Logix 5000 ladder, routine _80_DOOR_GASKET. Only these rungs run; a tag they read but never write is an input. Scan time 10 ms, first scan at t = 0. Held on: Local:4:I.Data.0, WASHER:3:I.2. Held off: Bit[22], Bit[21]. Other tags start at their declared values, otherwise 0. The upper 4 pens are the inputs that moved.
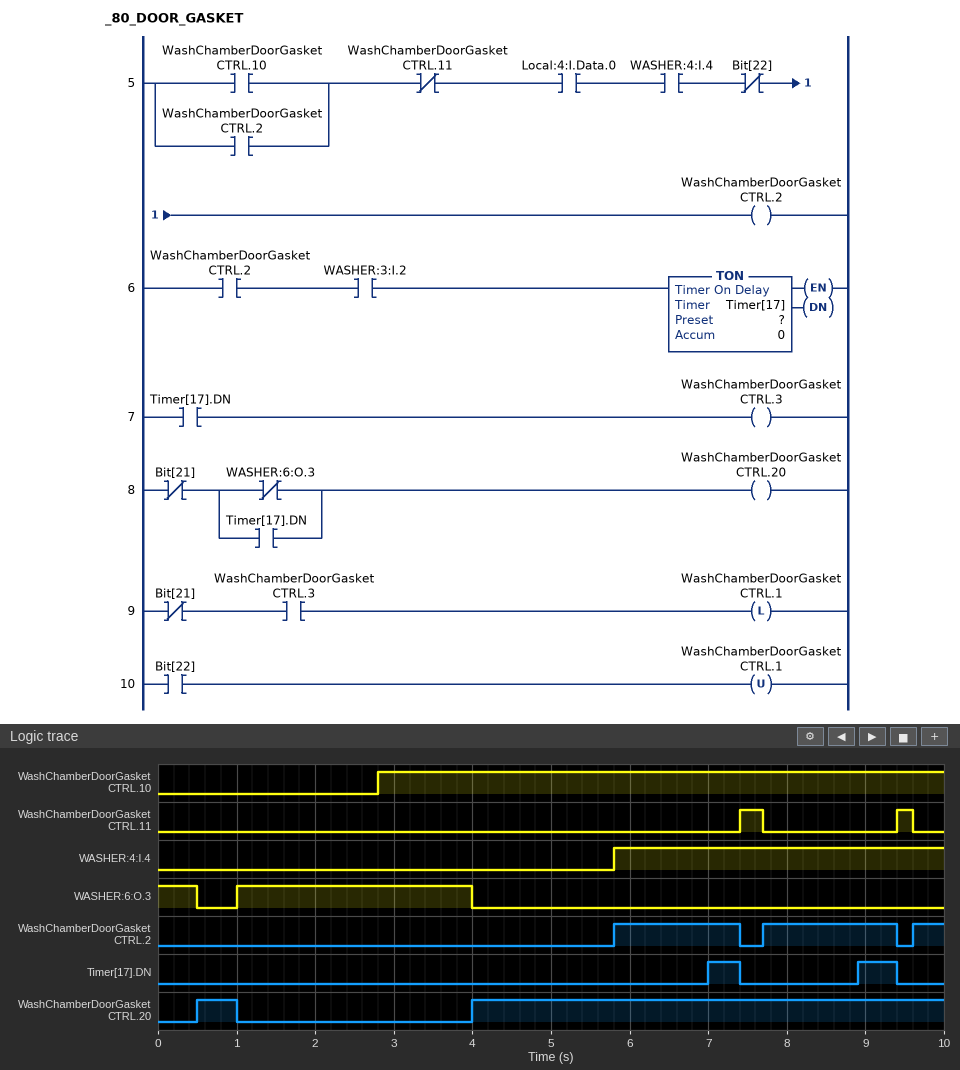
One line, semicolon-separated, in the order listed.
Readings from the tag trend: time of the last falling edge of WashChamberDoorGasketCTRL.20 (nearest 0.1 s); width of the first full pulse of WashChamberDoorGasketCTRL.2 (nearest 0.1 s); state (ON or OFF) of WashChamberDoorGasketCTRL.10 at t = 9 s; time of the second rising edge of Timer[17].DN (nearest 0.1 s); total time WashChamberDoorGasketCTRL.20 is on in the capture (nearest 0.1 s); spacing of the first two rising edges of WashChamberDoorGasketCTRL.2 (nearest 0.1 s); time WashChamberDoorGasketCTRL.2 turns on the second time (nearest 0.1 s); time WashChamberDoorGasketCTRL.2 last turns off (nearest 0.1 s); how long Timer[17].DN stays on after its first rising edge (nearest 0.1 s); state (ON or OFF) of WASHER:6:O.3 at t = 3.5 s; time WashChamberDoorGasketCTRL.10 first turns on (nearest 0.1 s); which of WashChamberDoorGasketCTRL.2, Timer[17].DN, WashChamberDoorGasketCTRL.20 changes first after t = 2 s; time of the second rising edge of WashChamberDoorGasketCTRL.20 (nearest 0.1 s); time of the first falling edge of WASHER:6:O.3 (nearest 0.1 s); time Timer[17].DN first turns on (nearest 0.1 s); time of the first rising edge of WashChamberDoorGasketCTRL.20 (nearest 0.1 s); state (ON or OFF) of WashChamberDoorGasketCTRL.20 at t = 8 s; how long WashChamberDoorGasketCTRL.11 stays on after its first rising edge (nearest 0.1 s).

1.0 s; 1.6 s; ON; 8.9 s; 6.5 s; 1.9 s; 7.7 s; 9.4 s; 0.4 s; ON; 2.8 s; WashChamberDoorGasketCTRL.20; 4.0 s; 0.5 s; 7.0 s; 0.5 s; ON; 0.3 s
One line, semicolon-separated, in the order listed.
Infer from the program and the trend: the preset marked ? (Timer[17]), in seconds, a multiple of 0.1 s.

1.2 s
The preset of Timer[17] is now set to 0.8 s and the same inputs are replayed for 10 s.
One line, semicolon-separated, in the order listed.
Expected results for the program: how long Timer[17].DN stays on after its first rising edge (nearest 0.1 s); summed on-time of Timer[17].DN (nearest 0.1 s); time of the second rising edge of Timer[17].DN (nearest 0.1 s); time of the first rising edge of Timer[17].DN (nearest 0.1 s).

0.8 s; 1.7 s; 8.5 s; 6.6 s
